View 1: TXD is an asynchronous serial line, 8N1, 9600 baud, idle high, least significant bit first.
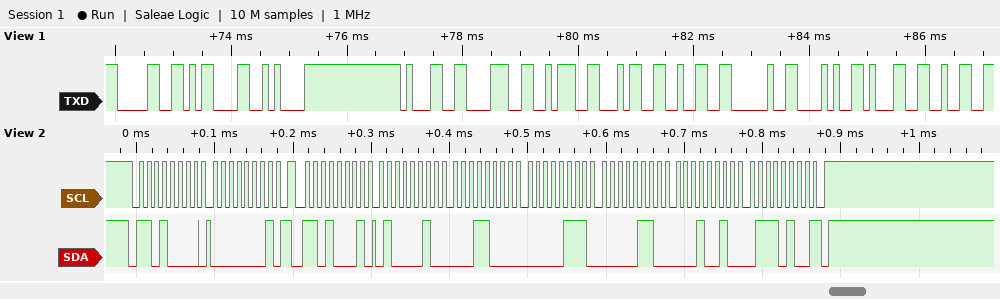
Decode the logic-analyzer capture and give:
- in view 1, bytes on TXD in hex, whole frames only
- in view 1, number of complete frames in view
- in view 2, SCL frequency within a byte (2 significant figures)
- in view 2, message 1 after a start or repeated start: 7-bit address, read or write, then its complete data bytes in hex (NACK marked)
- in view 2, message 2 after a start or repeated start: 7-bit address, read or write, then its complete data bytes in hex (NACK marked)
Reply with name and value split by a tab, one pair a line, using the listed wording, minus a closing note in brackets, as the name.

in view 1, bytes on TXD in hex, whole frames only	30 0D 0A 31 38 3A 34 32 20 28 31 32
in view 1, number of complete frames in view	12
in view 2, SCL frequency within a byte	100 kHz
in view 2, message 1 after a start or repeated start: 7-bit address, read or write, then its complete data bytes in hex	0x68 write: 01
in view 2, message 2 after a start or repeated start: 7-bit address, read or write, then its complete data bytes in hex	0x68 read: 42 18 07 06 12 74 NACK
